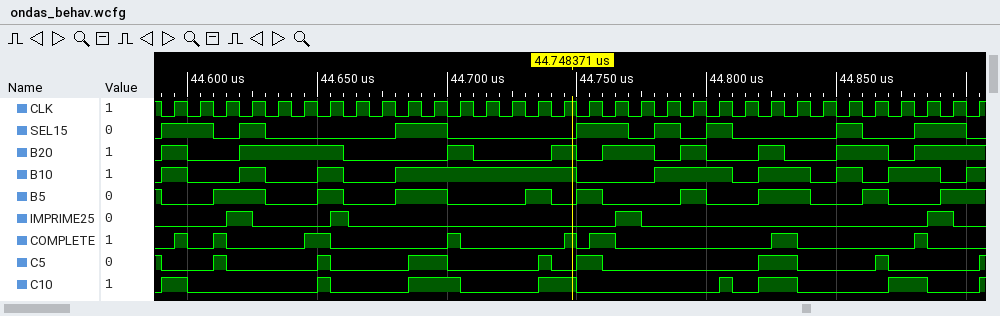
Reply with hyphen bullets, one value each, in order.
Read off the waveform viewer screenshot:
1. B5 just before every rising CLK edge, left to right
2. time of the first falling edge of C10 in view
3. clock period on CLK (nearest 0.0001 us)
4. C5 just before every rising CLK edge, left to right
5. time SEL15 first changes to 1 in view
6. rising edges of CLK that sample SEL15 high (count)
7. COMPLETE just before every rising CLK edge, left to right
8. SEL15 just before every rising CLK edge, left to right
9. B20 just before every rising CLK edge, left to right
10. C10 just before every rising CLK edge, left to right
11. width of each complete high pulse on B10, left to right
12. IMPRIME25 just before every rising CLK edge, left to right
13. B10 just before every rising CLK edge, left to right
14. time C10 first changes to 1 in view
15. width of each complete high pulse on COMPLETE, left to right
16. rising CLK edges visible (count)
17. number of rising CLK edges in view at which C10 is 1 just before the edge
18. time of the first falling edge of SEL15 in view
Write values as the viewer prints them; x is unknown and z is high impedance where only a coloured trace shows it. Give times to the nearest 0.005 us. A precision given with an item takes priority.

- 0 0 1 1 0 0 1 0 0 1 1 0 0 0 1 0 1 0 0 0 1 0 0 1 1 0 0 1 0 0 1 1
- 44.6 us
- 0.01 us
- 0 0 1 0 0 0 1 0 0 0 1 0 0 0 0 0 1 0 0 0 0 0 0 1 1 0 0 0 0 0 0 0
- 44.59 us
- 12
- 0 0 1 0 0 0 1 0 0 0 0 1 0 0 0 0 0 1 0 0 0 0 0 0 1 0 0 0 0 1 0 0
- 1 1 0 1 0 0 0 0 0 1 1 0 0 0 0 0 1 1 0 1 0 1 0 0 0 0 1 0 0 1 1 0
- 1 0 0 1 1 1 1 0 0 0 0 1 0 0 0 1 0 1 1 0 1 0 0 1 0 0 1 1 0 1 1 1
- 1 0 0 0 0 0 1 0 0 0 1 1 0 0 0 1 0 0 0 0 0 0 0 1 1 0 0 0 1 1 0 0
- 0.01 us, 0.01 us, 0.01 us, 0.07 us, 0.03 us, 0.02 us, 0.01 us, 0.02 us
- 0 0 0 1 0 0 0 0 0 0 0 0 0 0 0 0 0 0 1 0 0 0 0 0 0 0 0 0 0 0 1 0
- 1 0 0 1 0 0 1 0 0 1 1 1 1 1 1 1 0 0 0 1 1 1 0 1 1 0 1 0 1 1 0 1
- 44.59 us
- 0.005 us, 0.005 us, 0.01 us, 0.005 us, 0.005 us, 0.01 us, 0.01 us, 0.005 us
- 32
- 9
- 44.61 us
